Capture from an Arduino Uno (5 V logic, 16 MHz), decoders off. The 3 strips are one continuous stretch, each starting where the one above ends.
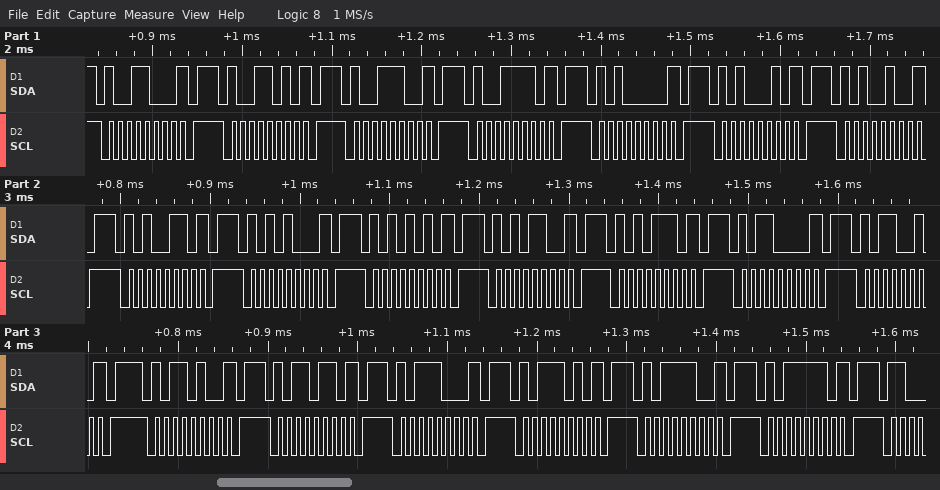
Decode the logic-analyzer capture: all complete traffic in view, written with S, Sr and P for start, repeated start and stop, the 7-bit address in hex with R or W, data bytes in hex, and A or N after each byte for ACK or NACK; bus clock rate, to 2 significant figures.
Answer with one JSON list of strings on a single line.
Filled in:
["S 4CW N P S 4DW N P S 4EW N P S 4FW N P S 50W N P S 51W N P S 52W N P S 53W N P S 54W N P S 55W N P S 56W N P S 57W N P S 58W N P S 59W N P S 5AW N P S 5BW N P S 5CW N P S 5DW N P S 5EW N P S 5FW N P", "100 kHz"]
